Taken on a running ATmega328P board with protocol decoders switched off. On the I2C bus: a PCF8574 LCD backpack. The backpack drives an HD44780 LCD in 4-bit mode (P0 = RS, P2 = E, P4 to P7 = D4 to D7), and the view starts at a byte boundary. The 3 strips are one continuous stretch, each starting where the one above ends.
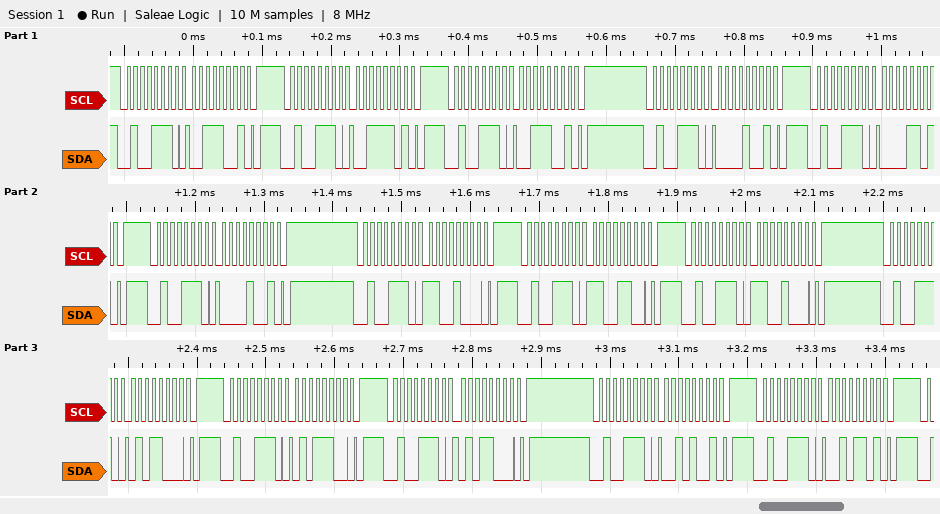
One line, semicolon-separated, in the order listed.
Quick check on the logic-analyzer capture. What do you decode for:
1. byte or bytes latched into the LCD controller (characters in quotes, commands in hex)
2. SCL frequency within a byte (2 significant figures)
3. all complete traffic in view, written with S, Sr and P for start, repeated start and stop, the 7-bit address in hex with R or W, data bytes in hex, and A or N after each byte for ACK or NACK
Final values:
'0' 0xC5; 100 kHz; S 27W A 39 A P S 27W A 3D A P S 27W A 39 A P S 27W A 09 A P S 27W A 0D A P S 27W A 09 A P S 27W A C8 A P S 27W A CC A P S 27W A C8 A P S 27W A 58 A P S 27W A 5C A P S 27W A 58 A P S 27W A 29 A P S 27W A 2D A P
